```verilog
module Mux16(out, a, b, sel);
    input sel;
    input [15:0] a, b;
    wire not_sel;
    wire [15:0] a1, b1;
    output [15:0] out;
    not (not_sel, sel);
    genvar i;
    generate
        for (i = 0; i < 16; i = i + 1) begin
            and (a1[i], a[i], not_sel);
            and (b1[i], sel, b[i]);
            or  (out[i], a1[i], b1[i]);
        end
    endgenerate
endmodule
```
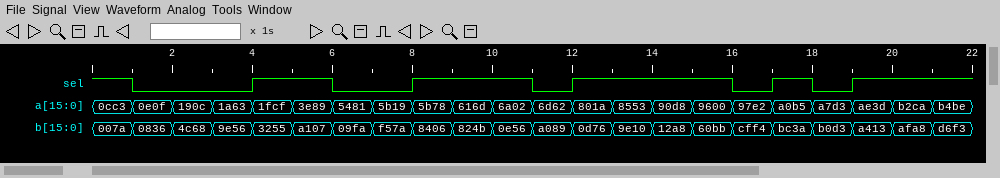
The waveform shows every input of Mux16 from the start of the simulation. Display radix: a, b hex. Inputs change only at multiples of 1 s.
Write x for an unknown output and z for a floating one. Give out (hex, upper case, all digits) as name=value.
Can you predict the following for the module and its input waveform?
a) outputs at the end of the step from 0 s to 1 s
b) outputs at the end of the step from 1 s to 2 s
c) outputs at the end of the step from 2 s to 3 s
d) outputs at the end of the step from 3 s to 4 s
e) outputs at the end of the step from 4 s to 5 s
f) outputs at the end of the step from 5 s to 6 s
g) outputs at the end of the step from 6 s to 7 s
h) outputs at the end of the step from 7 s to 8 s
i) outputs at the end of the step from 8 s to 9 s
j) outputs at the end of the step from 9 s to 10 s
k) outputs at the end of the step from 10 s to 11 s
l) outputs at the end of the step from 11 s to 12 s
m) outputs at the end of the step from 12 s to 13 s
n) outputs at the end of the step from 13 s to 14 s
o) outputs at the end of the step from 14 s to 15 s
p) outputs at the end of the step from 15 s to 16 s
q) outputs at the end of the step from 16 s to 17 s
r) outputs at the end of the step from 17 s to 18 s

out=007A
out=0E0F
out=190C
out=1A63
out=3255
out=A107
out=5481
out=5B19
out=8406
out=824B
out=0E56
out=6D62
out=0D76
out=9E10
out=12A8
out=60BB
out=97E2
out=BC3A
